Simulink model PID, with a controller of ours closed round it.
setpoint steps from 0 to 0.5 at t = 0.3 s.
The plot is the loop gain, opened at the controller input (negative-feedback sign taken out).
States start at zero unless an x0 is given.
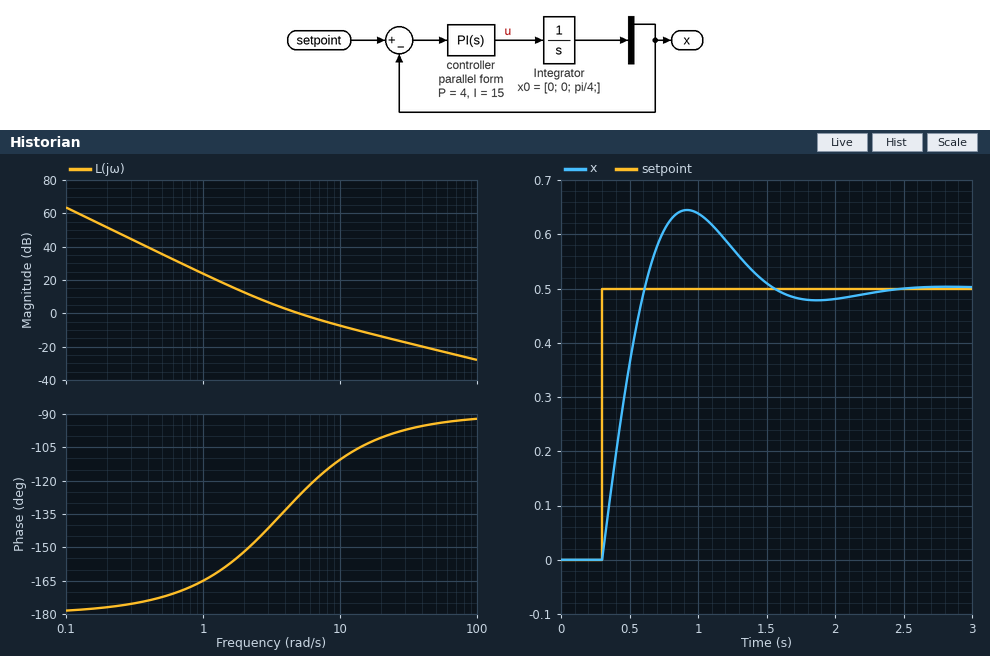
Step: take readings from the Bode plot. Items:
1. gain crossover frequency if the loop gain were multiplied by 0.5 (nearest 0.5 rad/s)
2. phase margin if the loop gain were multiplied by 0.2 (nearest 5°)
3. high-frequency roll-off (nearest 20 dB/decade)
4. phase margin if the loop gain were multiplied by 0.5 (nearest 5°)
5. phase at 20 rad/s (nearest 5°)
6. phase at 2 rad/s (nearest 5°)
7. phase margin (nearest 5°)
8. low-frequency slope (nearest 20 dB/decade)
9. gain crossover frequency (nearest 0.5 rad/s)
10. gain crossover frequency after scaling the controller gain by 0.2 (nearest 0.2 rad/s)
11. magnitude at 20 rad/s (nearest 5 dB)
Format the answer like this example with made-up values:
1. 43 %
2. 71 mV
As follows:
1. 3.0 rad/s
2. 25°
3. -20 dB/decade
4. 40°
5. -100°
6. -150°
7. 55°
8. -40 dB/decade
9. 5.0 rad/s
10. 1.8 rad/s
11. -15 dB
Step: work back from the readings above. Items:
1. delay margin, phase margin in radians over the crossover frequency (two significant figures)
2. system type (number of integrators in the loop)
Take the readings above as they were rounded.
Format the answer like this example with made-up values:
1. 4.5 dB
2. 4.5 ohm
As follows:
1. 0.19 s
2. 2
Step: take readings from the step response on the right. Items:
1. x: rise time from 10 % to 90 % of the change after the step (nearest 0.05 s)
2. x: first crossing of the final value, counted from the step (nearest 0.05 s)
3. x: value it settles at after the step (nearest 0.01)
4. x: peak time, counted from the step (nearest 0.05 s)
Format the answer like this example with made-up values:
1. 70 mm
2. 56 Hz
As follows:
1. 0.25 s
2. 0.30 s
3. 0.50
4. 0.60 s
